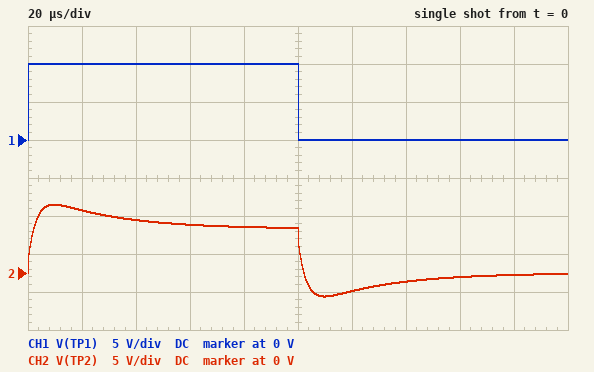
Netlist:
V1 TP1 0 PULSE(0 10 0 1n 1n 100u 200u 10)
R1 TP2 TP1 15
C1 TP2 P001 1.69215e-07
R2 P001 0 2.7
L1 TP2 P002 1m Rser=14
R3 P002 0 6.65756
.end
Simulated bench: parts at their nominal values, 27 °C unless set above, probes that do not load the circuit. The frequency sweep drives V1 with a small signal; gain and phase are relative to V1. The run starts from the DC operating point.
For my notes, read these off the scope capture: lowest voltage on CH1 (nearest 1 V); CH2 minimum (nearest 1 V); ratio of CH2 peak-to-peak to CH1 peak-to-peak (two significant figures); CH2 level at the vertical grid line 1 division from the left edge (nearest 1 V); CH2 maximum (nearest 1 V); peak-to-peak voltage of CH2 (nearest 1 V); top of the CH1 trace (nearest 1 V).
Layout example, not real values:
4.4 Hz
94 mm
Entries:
0 V
-3 V
1.2
8 V
9 V
12 V
10 V
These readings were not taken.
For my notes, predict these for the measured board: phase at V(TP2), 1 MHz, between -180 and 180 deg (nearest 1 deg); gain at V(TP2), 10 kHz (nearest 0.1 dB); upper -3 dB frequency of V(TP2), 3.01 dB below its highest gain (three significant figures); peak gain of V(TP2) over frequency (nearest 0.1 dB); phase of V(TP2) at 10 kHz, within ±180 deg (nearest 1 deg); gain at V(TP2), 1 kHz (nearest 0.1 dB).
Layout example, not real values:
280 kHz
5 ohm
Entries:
-16 deg
-0.6 dB
61.3 kHz
-0.4 dB
3 deg
-4.5 dB
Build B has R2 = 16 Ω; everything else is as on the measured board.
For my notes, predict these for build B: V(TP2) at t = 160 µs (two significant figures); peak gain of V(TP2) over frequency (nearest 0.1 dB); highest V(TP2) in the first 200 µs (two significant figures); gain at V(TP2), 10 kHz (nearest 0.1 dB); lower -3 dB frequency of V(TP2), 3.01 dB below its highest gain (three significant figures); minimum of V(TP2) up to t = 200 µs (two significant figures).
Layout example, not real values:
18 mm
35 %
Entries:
-550 mV
-0.7 dB
8.5 V
-0.8 dB
2.16 kHz
-2.6 V
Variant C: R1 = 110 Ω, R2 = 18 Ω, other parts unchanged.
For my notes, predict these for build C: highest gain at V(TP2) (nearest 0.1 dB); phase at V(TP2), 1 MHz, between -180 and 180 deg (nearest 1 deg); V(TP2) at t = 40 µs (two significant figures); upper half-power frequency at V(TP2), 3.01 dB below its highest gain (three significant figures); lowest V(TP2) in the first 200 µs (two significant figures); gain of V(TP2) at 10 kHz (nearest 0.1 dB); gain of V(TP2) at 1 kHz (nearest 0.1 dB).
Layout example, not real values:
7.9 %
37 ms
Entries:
-4.5 dB
-2 deg
2.1 V
21.0 kHz
-2.4 V
-5.1 dB
-15.6 dB
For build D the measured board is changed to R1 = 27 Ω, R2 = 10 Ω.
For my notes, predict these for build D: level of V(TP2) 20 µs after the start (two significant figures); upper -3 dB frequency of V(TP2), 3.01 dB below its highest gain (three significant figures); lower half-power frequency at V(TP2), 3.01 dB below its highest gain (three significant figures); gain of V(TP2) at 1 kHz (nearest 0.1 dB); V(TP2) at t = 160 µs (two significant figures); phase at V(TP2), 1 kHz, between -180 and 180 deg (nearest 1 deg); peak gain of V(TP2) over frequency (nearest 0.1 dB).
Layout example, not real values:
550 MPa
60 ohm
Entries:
7.3 V
37.3 kHz
4.13 kHz
-6.9 dB
-380 mV
9 deg
-1.1 dB
